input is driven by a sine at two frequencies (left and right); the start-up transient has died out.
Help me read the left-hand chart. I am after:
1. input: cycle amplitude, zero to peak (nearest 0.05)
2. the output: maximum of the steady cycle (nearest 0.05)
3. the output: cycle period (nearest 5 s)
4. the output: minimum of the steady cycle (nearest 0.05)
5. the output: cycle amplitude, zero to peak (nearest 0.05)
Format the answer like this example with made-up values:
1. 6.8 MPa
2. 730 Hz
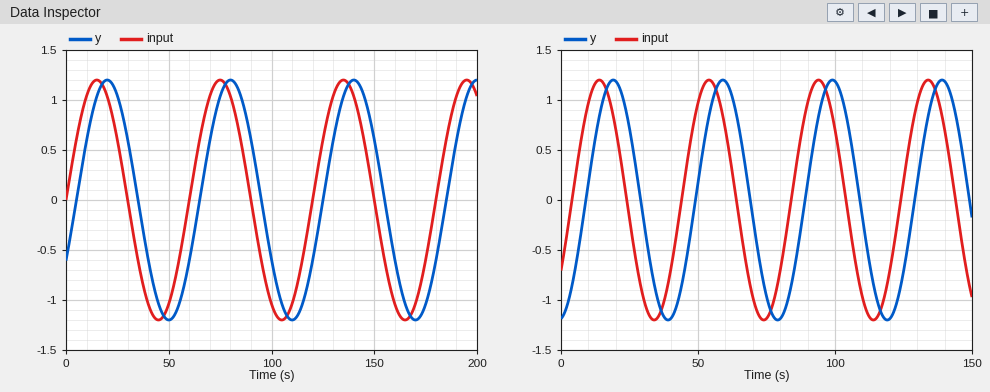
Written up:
1. 1.20
2. 1.20
3. 60 s
4. -1.20
5. 1.20
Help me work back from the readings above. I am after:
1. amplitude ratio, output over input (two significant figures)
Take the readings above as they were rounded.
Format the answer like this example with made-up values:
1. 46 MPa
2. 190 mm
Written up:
1. 1.0
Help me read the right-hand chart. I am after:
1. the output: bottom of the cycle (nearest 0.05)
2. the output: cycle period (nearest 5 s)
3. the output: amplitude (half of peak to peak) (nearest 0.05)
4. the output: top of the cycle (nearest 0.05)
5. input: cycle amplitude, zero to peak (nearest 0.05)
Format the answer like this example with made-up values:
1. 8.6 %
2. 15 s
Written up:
1. -1.20
2. 40 s
3. 1.20
4. 1.20
5. 1.20
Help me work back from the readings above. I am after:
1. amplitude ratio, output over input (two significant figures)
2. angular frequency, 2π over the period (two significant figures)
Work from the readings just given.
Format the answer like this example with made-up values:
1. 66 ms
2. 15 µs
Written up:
1. 1.0
2. 0.16 rad/s
